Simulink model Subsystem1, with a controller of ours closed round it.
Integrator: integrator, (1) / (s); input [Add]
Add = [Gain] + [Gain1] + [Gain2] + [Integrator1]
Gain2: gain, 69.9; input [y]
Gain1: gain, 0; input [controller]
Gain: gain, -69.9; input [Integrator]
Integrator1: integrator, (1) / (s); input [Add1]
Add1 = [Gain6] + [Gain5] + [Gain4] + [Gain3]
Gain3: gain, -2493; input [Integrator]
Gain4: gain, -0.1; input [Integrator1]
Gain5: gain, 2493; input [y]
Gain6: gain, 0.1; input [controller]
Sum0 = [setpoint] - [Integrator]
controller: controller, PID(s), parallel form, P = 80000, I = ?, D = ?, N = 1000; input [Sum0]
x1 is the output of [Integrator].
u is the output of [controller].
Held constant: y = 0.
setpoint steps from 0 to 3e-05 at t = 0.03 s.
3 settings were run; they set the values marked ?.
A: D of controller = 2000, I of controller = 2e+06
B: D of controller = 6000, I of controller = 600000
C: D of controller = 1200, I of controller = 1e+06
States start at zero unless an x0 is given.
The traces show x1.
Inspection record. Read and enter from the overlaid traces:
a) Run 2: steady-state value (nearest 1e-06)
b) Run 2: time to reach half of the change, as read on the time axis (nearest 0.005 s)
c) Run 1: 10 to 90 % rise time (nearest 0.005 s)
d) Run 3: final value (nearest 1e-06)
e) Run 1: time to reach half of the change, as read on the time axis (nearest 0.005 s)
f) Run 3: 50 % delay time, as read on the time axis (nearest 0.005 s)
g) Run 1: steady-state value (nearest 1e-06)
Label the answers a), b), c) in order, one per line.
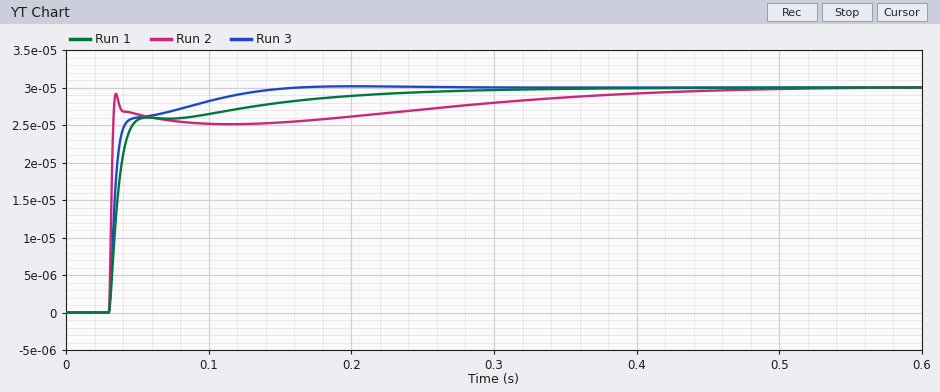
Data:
a) 0.000030
b) 0.030 s
c) 0.085 s
d) 0.000030
e) 0.035 s
f) 0.035 s
g) 0.000030
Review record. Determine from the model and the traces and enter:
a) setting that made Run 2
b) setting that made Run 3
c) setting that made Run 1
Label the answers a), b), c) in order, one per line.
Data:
a) B
b) A
c) C
